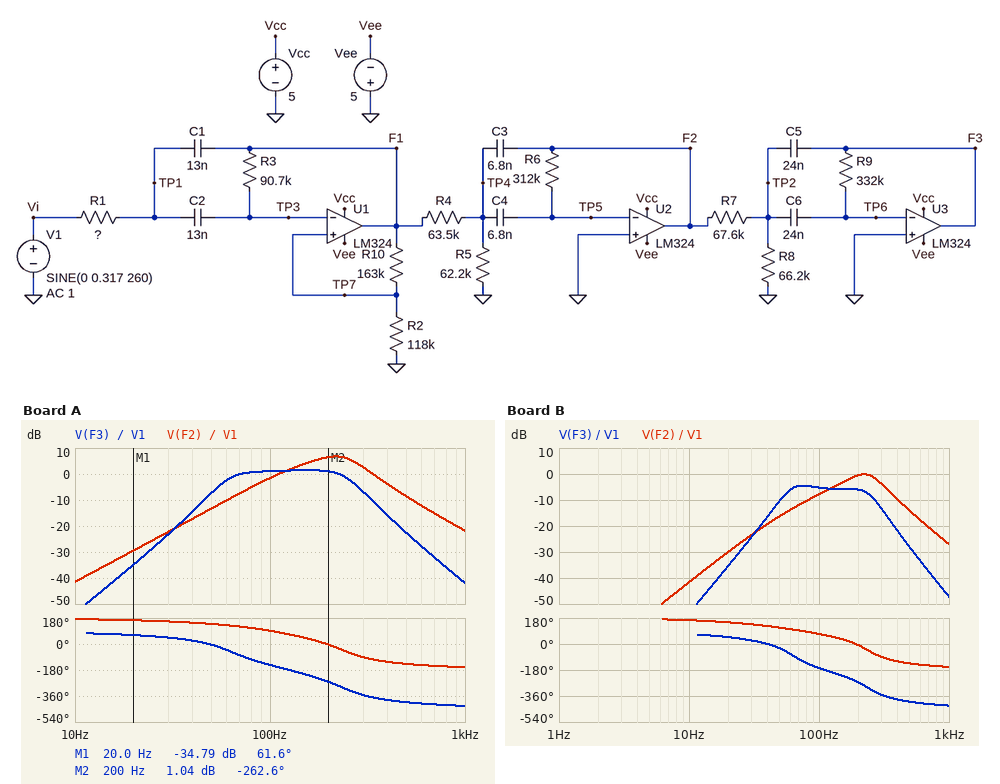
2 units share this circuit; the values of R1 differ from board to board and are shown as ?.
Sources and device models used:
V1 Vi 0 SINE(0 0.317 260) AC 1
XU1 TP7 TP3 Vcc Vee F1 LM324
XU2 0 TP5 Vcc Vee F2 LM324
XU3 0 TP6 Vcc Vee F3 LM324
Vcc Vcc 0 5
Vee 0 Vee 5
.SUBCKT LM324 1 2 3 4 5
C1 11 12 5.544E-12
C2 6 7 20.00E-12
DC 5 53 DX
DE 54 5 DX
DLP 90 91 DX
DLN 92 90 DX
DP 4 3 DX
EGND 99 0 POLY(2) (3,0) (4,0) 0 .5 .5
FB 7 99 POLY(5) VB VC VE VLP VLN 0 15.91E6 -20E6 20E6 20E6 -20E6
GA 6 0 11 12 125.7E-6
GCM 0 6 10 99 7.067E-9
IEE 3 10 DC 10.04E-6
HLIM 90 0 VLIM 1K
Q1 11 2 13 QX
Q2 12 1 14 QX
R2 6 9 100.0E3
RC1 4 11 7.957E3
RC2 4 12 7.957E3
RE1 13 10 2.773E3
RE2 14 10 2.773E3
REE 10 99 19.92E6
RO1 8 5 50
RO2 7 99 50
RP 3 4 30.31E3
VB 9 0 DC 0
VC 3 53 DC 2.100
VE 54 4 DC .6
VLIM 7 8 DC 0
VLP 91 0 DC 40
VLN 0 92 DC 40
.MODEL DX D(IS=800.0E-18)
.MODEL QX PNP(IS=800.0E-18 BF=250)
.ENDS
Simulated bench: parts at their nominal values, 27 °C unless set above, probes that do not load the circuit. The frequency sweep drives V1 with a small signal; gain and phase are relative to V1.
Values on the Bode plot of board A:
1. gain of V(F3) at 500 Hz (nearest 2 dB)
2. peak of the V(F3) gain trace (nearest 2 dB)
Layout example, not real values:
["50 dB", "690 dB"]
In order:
["-22 dB", "2 dB"]
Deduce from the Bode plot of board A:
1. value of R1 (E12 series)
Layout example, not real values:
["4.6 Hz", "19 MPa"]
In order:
["100 kΩ"]
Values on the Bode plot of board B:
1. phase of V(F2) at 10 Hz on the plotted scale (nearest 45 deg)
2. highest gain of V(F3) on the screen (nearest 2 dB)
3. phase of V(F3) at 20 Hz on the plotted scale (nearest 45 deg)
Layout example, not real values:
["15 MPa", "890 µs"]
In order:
["180 deg", "-4 dB", "45 deg"]
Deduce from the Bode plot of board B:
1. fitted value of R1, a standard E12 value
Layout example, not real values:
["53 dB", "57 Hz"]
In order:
["180 kΩ"]
